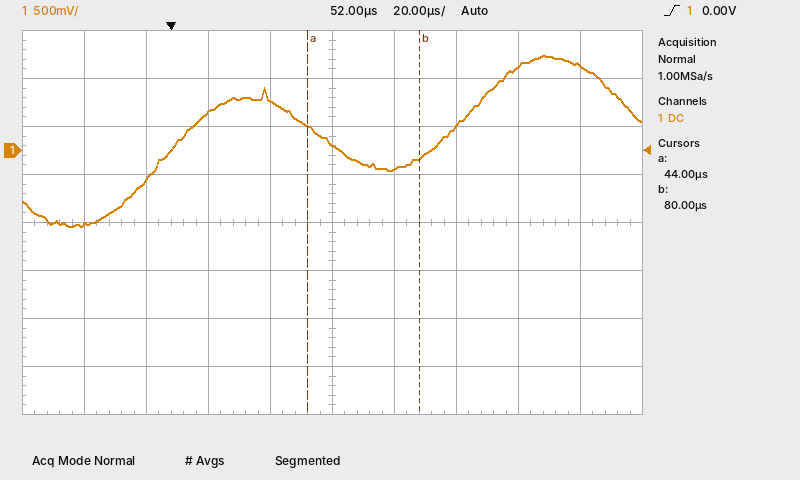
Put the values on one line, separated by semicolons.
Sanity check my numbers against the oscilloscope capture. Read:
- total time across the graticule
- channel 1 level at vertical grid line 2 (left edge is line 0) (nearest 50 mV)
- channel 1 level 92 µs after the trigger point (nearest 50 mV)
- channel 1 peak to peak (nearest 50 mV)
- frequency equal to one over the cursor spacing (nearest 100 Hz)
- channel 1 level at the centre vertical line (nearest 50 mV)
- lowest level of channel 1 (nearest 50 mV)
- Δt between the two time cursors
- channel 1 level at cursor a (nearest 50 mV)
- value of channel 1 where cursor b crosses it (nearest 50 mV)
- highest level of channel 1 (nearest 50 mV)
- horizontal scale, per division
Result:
200 µs; -300 mV; 250 mV; 1.80 V; 27.8 kHz; 50 mV; -800 mV; 36 µs; 250 mV; -50 mV; 1.00 V; 20 µs
